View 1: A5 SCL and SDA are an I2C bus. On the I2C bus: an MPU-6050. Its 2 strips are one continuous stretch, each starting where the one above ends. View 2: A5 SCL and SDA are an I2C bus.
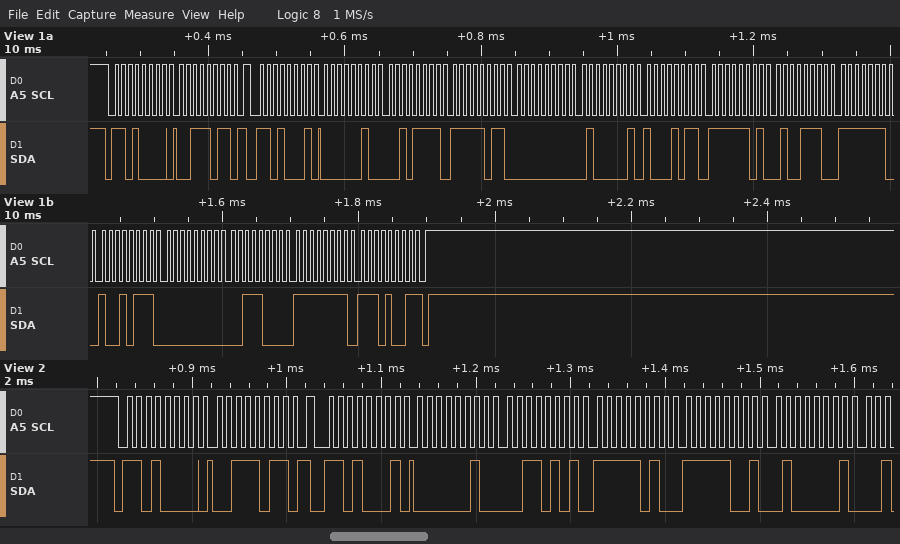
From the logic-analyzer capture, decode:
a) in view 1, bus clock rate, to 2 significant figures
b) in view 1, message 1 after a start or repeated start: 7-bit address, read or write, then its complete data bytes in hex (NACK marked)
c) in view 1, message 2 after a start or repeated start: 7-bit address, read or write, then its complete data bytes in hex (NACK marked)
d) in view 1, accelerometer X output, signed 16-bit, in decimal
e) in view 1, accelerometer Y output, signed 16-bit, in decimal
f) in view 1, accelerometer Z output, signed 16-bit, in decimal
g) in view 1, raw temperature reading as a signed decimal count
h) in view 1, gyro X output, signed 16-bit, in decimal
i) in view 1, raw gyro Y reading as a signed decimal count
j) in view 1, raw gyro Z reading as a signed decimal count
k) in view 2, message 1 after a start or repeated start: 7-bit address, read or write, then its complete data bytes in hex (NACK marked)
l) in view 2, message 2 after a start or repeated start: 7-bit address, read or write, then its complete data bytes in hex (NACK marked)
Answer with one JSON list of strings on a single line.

["100 kHz", "0x68 write: 3B", "0x68 read: 02 2F FB 00 41 8B FD 4E FE 97 00 38 FF E9 NACK", "559", "-1280", "16779", "-690", "-361", "56", "-23", "0x68 write: 3B", "0x68 read: 02 35 FA F9 41"]
